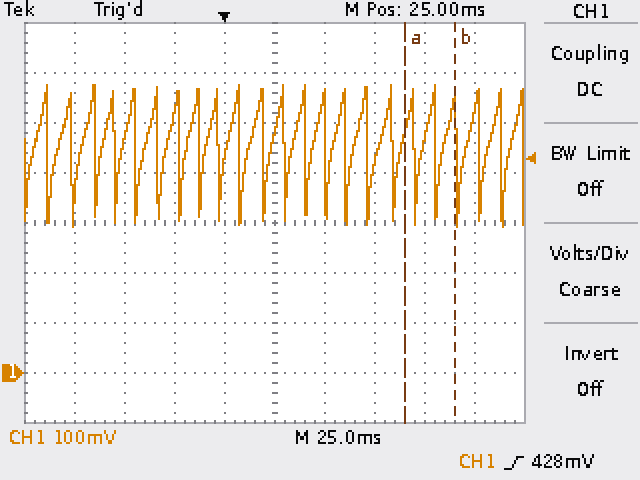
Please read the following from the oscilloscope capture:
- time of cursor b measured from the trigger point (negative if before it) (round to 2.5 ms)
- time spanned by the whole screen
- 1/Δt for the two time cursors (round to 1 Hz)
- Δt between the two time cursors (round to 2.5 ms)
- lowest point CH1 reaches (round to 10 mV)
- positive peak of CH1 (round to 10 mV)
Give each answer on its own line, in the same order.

+115.0 ms
250 ms
40 Hz
25.0 ms
290 mV
580 mV
